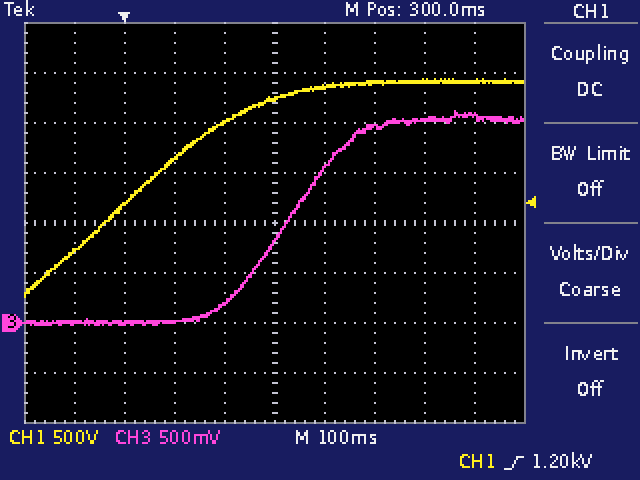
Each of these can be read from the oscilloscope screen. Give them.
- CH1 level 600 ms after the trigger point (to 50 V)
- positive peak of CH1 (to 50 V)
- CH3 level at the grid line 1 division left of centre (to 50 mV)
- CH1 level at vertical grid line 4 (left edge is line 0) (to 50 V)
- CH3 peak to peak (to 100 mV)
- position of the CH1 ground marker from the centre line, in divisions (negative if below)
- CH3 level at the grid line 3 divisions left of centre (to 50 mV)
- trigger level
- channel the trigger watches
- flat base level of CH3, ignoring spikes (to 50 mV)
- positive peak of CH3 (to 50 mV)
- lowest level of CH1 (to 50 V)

2.40 kV
2.45 kV
200 mV
2.00 kV
2.10 V
-2.0 div
0 mV
1.20 kV
CH1
0 mV
2.10 V
250 V
